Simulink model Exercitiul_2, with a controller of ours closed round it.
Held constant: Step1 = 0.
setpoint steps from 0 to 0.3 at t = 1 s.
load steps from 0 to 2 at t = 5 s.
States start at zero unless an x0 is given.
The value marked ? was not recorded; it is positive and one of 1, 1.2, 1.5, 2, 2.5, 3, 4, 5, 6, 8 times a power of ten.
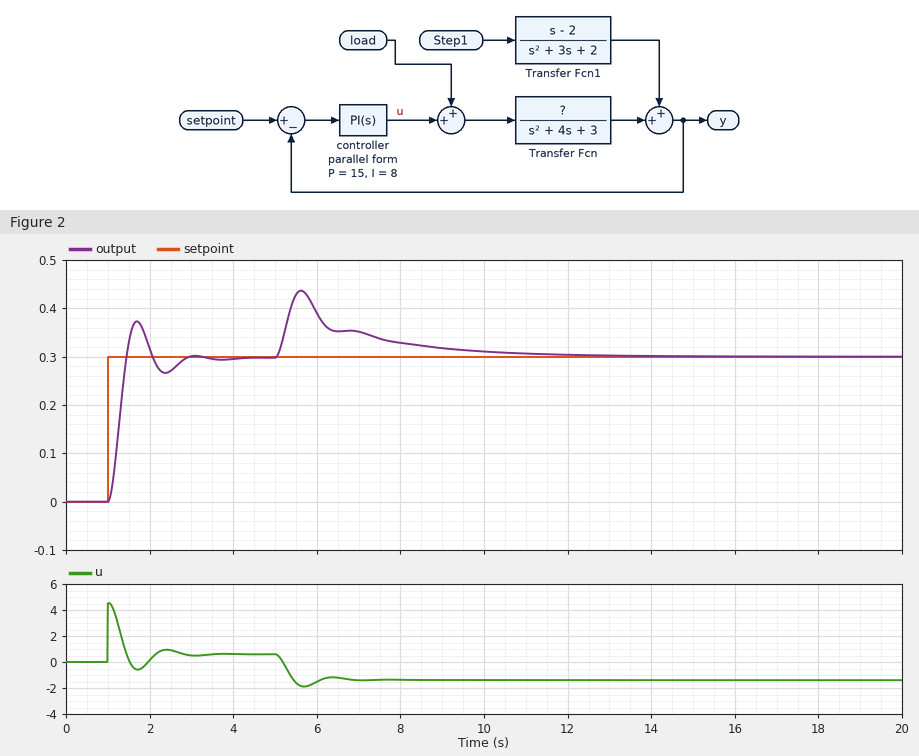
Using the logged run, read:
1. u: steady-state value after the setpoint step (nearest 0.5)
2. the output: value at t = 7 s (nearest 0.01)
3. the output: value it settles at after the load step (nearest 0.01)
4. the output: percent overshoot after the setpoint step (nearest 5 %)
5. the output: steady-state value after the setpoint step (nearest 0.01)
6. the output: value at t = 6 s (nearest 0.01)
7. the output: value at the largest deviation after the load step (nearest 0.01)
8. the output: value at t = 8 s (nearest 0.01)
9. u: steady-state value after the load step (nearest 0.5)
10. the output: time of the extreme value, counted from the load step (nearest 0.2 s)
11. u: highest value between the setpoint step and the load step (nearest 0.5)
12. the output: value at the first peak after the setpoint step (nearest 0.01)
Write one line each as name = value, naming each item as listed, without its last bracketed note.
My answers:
u: steady-state value after the setpoint step = 0.5
the output: value at t = 7 s = 0.35
the output: value it settles at after the load step = 0.30
the output: percent overshoot after the setpoint step = 25 %
the output: steady-state value after the setpoint step = 0.30
the output: value at t = 6 s = 0.39
the output: value at the largest deviation after the load step = 0.44
the output: value at t = 8 s = 0.33
u: steady-state value after the load step = -1.5
the output: time of the extreme value, counted from the load step = 0.6 s
u: highest value between the setpoint step and the load step = 4.5
the output: value at the first peak after the setpoint step = 0.37
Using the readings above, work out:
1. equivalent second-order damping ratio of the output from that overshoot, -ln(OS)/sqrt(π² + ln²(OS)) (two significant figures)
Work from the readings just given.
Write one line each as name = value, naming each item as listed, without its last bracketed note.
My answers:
equivalent second-order damping ratio of the output from that overshoot, -ln(OS)/sqrt(π² + ln²(OS)) = 0.40
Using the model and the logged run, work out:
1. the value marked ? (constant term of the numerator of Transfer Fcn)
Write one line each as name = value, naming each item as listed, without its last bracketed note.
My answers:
the value marked ? = 1.5
